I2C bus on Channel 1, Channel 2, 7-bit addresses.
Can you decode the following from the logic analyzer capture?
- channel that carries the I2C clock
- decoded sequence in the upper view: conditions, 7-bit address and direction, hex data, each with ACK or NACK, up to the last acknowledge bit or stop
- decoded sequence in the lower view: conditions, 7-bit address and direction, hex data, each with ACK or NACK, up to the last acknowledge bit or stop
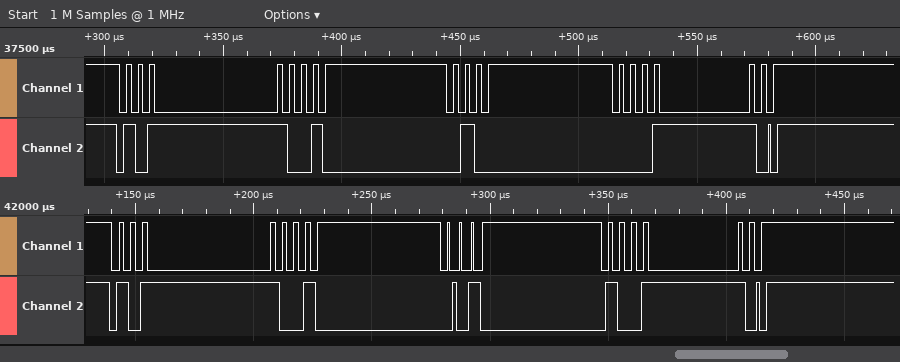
Channel 1
start, address 59 write ACK, 83 ACK, stop
start, address 59 write ACK, 53 ACK, stop
